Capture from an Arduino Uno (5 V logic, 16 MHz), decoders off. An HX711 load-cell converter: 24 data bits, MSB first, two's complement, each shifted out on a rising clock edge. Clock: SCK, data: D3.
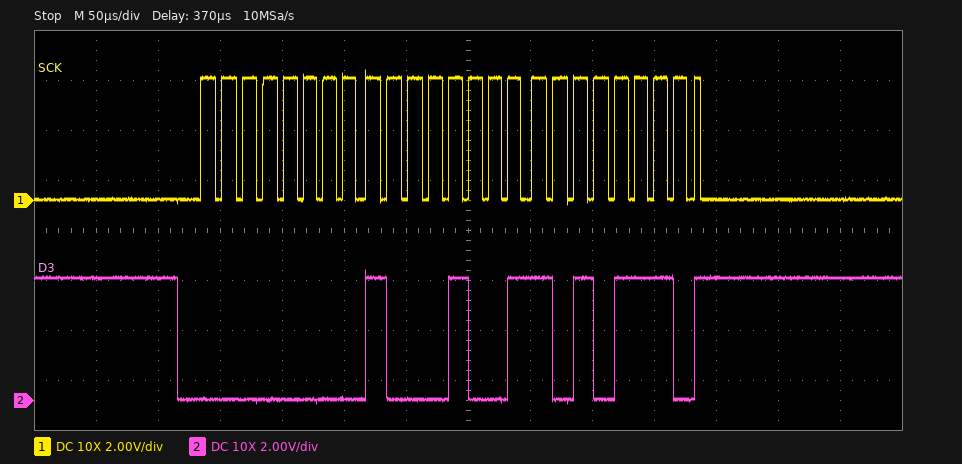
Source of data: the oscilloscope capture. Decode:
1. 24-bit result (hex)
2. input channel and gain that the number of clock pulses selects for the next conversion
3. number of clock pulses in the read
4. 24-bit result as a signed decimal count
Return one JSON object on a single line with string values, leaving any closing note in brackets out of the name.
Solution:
{"24-bit result": "0x0089AE", "input channel and gain that the number of clock pulses selects for the next conversion": "channel A, gain 128", "number of clock pulses in the read": "25", "24-bit result as a signed decimal count": "35246"}
